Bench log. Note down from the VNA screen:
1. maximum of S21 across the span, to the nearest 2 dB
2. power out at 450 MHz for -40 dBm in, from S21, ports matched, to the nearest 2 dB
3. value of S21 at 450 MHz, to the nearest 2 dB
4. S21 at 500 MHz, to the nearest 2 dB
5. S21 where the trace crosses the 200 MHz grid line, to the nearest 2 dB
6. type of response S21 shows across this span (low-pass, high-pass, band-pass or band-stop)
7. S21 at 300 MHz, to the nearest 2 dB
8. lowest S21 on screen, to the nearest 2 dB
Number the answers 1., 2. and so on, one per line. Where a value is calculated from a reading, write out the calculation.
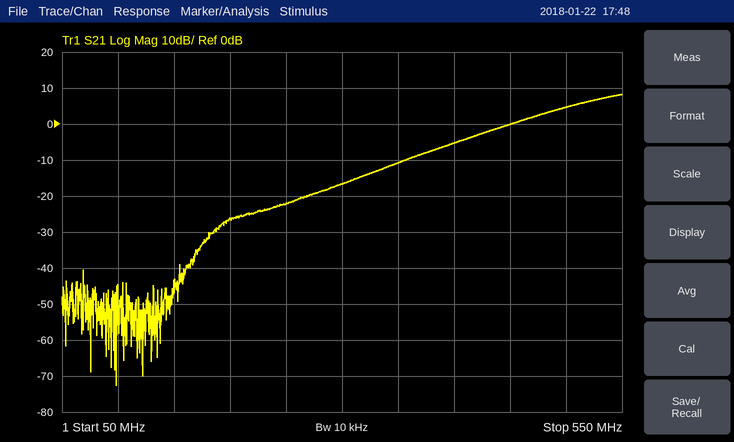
1. 8 dB
2. -40 dBm + (0 dB) = -40 dBm
3. 0 dB
4. 4 dB
5. -26 dB
6. high-pass
7. -16 dB
8. -72 dB
